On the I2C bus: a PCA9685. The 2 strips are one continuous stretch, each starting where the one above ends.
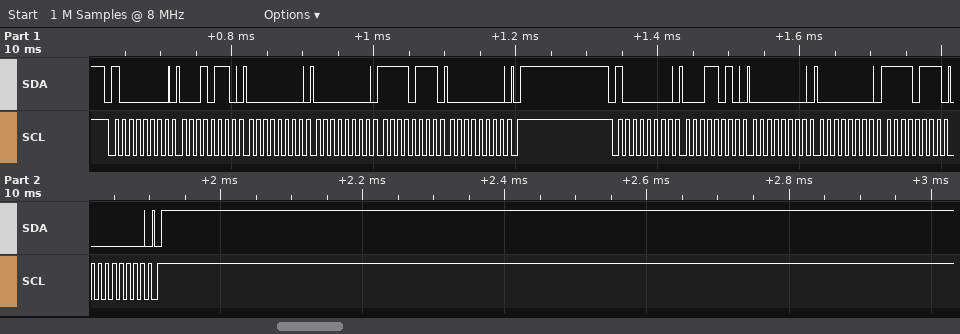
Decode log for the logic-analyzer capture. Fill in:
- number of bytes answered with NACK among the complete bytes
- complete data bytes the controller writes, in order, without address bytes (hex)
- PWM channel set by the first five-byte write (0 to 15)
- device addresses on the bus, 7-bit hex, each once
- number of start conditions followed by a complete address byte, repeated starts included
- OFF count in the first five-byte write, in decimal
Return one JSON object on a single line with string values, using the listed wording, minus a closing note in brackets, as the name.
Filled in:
{"number of bytes answered with NACK among the complete bytes": "0", "complete data bytes the controller writes, in order, without address bytes": "16 00 00 F7 00 1A 00 00 F7 00", "PWM channel set by the first five-byte write": "4", "device addresses on the bus, 7-bit hex, each once": "0x40", "number of start conditions followed by a complete address byte, repeated starts included": "2", "OFF count in the first five-byte write, in decimal": "247"}
